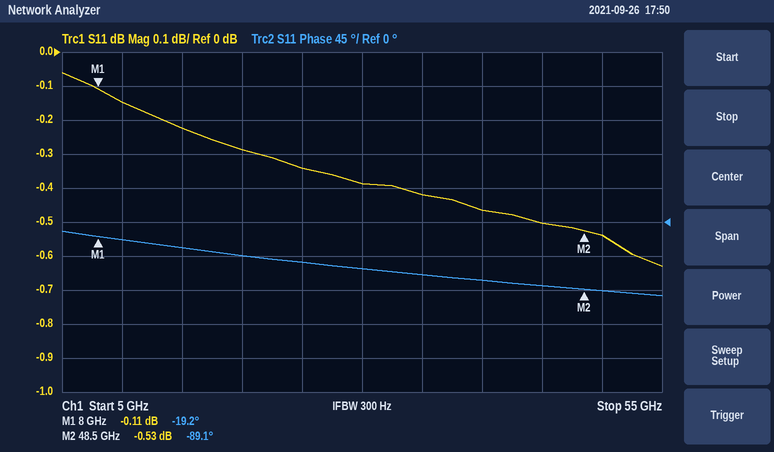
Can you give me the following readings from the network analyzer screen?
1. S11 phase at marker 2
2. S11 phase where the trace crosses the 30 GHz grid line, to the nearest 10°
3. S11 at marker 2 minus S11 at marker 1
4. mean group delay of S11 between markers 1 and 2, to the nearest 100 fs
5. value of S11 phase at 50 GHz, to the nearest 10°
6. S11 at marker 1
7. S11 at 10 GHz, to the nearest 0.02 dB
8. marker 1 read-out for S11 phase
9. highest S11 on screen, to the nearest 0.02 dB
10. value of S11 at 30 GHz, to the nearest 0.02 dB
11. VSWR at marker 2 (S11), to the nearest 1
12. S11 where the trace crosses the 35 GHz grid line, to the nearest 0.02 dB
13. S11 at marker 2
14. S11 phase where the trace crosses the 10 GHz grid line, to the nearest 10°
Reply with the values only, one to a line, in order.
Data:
-89.1°
-60°
-0.42 dB
4.8 ps
-90°
-0.11 dB
-0.14 dB
-19.2°
-0.06 dB
-0.38 dB
33
-0.42 dB
-0.53 dB
-20°
